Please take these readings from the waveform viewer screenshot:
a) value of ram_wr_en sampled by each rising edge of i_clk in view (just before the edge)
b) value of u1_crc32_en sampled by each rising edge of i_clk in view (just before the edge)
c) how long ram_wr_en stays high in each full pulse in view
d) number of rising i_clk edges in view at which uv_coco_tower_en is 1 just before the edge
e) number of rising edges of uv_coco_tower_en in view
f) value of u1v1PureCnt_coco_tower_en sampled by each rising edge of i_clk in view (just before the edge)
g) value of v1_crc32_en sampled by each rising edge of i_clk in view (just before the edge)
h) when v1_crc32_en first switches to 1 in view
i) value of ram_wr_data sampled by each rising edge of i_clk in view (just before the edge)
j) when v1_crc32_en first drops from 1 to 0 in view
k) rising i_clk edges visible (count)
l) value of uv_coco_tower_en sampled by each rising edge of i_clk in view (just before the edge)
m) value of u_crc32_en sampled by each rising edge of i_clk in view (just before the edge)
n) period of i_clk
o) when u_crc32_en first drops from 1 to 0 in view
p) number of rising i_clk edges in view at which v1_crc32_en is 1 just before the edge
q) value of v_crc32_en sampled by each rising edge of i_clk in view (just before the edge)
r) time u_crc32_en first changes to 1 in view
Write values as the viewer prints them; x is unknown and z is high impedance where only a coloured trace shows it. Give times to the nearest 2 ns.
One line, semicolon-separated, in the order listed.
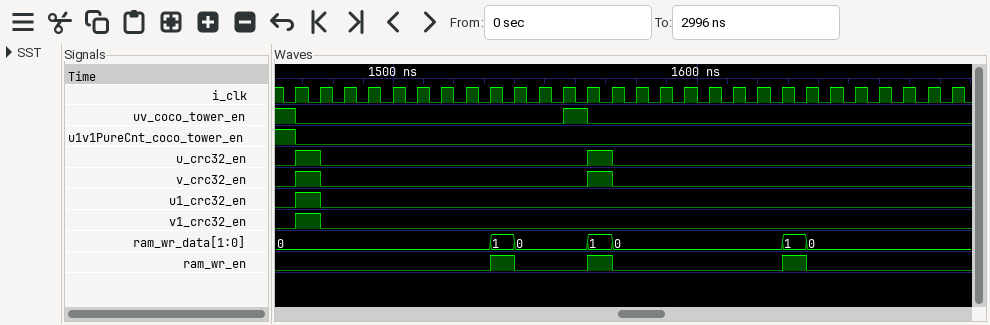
0 0 0 0 0 0 0 0 0 1 0 0 0 1 0 0 0 0 0 0 0 1 0 0 0 0 0 0; 0 1 0 0 0 0 0 0 0 0 0 0 0 0 0 0 0 0 0 0 0 0 0 0 0 0 0 0; 8 ns, 8 ns, 8 ns; 2; 1; 1 0 0 0 0 0 0 0 0 0 0 0 0 0 0 0 0 0 0 0 0 0 0 0 0 0 0 0; 0 1 0 0 0 0 0 0 0 0 0 0 0 0 0 0 0 0 0 0 0 0 0 0 0 0 0 0; 1468 ns; 0, 0, 0, 0, 0, 0, 0, 0, 0, 1, 0, 0, 0, 1, 0, 0, 0, 0, 0, 0, 0, 1, 0, 0, 0, 0, 0, 0; 1476 ns; 28; 1 0 0 0 0 0 0 0 0 0 0 0 1 0 0 0 0 0 0 0 0 0 0 0 0 0 0 0; 0 1 0 0 0 0 0 0 0 0 0 0 0 1 0 0 0 0 0 0 0 0 0 0 0 0 0 0; 8 ns; 1476 ns; 1; 0 1 0 0 0 0 0 0 0 0 0 0 0 1 0 0 0 0 0 0 0 0 0 0 0 0 0 0; 1468 ns
